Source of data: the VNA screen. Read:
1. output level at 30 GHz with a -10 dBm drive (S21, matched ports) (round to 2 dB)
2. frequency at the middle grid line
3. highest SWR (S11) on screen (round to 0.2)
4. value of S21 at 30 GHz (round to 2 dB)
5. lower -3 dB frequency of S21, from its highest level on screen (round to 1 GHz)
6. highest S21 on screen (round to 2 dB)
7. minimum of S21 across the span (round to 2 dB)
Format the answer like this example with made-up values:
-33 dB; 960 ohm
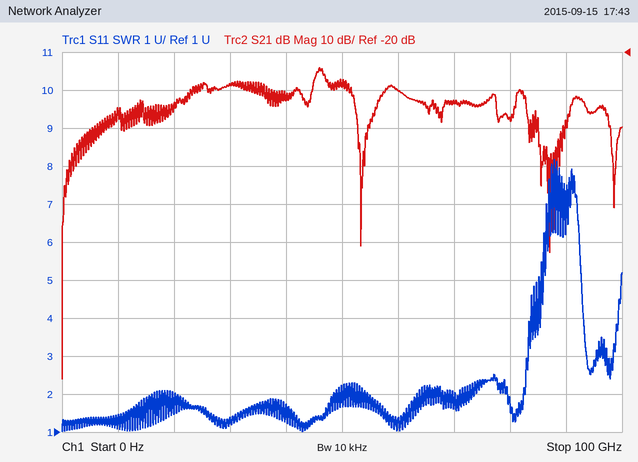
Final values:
-38 dBm; 50 GHz; 8.2; -28 dB; 45 GHz; -24 dB; -106 dB
